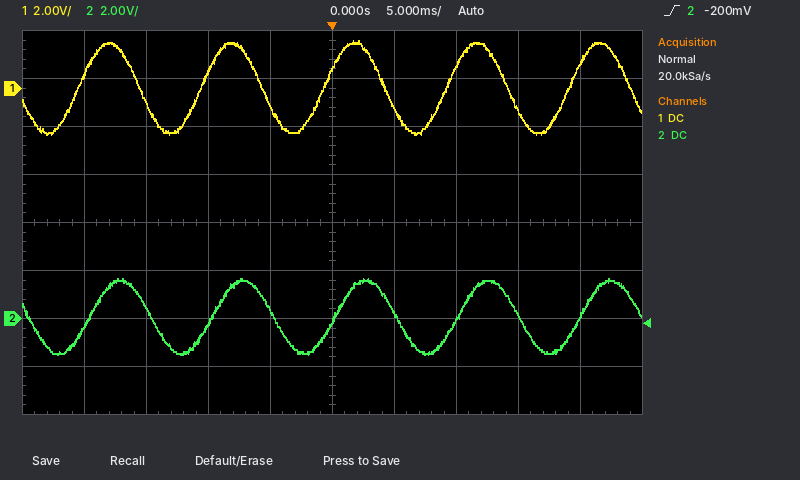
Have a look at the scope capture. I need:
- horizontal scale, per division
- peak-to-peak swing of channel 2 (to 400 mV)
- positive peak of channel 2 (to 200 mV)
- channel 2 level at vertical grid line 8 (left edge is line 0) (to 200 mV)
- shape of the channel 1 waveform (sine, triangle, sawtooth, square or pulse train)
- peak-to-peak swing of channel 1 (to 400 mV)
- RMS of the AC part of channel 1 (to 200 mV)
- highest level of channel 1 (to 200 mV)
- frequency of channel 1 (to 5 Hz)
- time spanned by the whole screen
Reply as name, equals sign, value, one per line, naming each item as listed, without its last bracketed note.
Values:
horizontal scale, per division = 5 ms
peak-to-peak swing of channel 2 = 3.2 V
positive peak of channel 2 = 1.6 V
channel 2 level at vertical grid line 8 (left edge is line 0) = 200 mV
shape of the channel 1 waveform = sine
peak-to-peak swing of channel 1 = 4.0 V
RMS of the AC part of channel 1 = 1.4 V
highest level of channel 1 = 2.0 V
frequency of channel 1 = 100 Hz
time spanned by the whole screen = 50 ms
